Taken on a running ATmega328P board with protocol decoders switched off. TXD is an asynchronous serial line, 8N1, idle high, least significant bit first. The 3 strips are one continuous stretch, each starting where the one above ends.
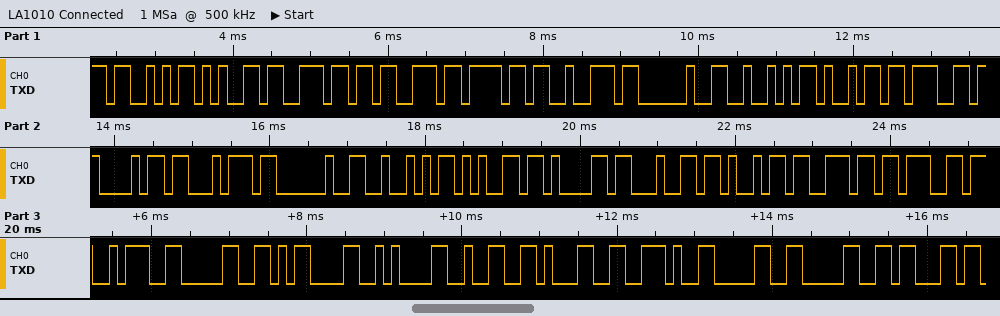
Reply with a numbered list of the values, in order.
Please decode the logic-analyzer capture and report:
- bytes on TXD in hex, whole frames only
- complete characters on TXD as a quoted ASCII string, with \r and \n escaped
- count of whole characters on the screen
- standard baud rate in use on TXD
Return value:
1. 53 65 6E 73 6F 72 20 52 69 67 68 74 20 52 65 61 64 69 6E 67 3A 30 0D 0A 32 31 2E 30 30 63
2. "Sensor Right Reading:0\r\n21.00c"
3. 30
4. 9600 baud
